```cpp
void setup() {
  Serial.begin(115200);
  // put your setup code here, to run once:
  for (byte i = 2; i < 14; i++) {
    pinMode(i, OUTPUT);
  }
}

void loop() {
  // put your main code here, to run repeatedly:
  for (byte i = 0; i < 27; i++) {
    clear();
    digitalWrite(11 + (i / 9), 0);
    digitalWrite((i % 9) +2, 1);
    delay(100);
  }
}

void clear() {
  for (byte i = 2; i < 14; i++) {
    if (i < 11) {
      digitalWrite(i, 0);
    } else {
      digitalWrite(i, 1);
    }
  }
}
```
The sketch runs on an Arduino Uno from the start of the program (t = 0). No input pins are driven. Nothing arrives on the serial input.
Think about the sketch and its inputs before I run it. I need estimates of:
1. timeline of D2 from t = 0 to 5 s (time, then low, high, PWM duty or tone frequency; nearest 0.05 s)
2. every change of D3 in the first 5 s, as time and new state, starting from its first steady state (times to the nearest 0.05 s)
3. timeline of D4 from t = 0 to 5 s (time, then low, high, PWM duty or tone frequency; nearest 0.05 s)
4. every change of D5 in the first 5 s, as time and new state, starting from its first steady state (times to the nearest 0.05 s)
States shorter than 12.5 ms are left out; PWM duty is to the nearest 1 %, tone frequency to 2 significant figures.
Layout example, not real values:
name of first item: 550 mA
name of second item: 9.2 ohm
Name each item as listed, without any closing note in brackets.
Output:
timeline of D2 from t = 0 to 5 s: 0 s high; 0.1 s low; 0.9 s high; 1 s low; 1.8 s high; 1.9 s low; 2.7 s high; 2.8 s low; 3.6 s high; 3.7 s low; 4.5 s high; 4.6 s low
every change of D3 in the first 5 s, as time and new state, starting from its first steady state: 0 s low; 0.1 s high; 0.2 s low; 1 s high; 1.1 s low; 1.9 s high; 2 s low; 2.8 s high; 2.9 s low; 3.7 s high; 3.8 s low; 4.6 s high; 4.7 s low
timeline of D4 from t = 0 to 5 s: 0 s low; 0.2 s high; 0.3 s low; 1.1 s high; 1.2 s low; 2 s high; 2.1 s low; 2.9 s high; 3 s low; 3.8 s high; 3.9 s low; 4.7 s high; 4.8 s low
every change of D5 in the first 5 s, as time and new state, starting from its first steady state: 0 s low; 0.3 s high; 0.4 s low; 1.2 s high; 1.3 s low; 2.1 s high; 2.2 s low; 3 s high; 3.1 s low; 3.9 s high; 4 s low; 4.8 s high; 4.9 s low
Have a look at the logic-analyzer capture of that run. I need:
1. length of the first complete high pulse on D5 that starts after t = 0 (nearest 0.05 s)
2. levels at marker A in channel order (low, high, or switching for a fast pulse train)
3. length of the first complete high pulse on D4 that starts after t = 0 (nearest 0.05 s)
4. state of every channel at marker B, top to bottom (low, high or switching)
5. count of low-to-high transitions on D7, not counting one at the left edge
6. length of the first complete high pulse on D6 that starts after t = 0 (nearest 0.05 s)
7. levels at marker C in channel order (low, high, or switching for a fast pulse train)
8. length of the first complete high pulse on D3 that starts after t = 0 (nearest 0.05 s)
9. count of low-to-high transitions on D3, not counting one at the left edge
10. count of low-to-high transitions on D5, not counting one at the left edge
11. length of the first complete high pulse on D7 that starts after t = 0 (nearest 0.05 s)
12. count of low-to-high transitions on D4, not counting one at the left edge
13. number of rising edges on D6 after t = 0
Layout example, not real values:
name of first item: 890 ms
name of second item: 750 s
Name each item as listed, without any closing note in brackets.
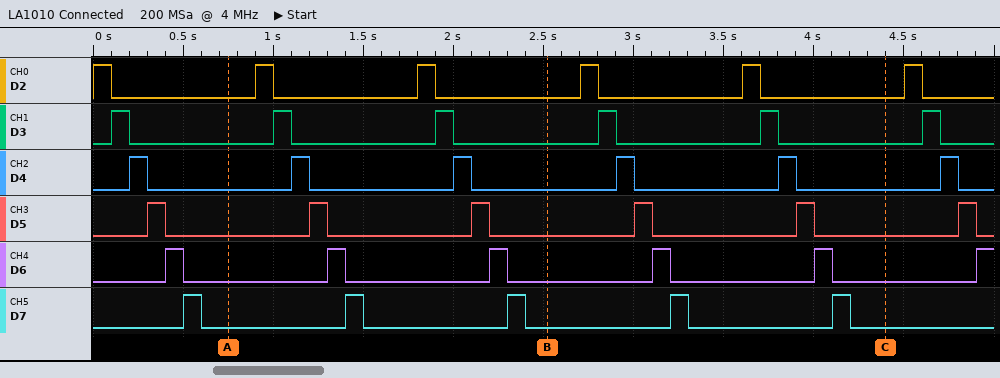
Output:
length of the first complete high pulse on D5 that starts after t = 0: 0.10 s
levels at marker A in channel order: D2 low, D3 low, D4 low, D5 low, D6 low, D7 low
length of the first complete high pulse on D4 that starts after t = 0: 0.10 s
state of every channel at marker B, top to bottom: D2 low, D3 low, D4 low, D5 low, D6 low, D7 low
count of low-to-high transitions on D7, not counting one at the left edge: 5
length of the first complete high pulse on D6 that starts after t = 0: 0.10 s
levels at marker C in channel order: D2 low, D3 low, D4 low, D5 low, D6 low, D7 low
length of the first complete high pulse on D3 that starts after t = 0: 0.10 s
count of low-to-high transitions on D3, not counting one at the left edge: 6
count of low-to-high transitions on D5, not counting one at the left edge: 6
length of the first complete high pulse on D7 that starts after t = 0: 0.10 s
count of low-to-high transitions on D4, not counting one at the left edge: 6
number of rising edges on D6 after t = 0: 6
